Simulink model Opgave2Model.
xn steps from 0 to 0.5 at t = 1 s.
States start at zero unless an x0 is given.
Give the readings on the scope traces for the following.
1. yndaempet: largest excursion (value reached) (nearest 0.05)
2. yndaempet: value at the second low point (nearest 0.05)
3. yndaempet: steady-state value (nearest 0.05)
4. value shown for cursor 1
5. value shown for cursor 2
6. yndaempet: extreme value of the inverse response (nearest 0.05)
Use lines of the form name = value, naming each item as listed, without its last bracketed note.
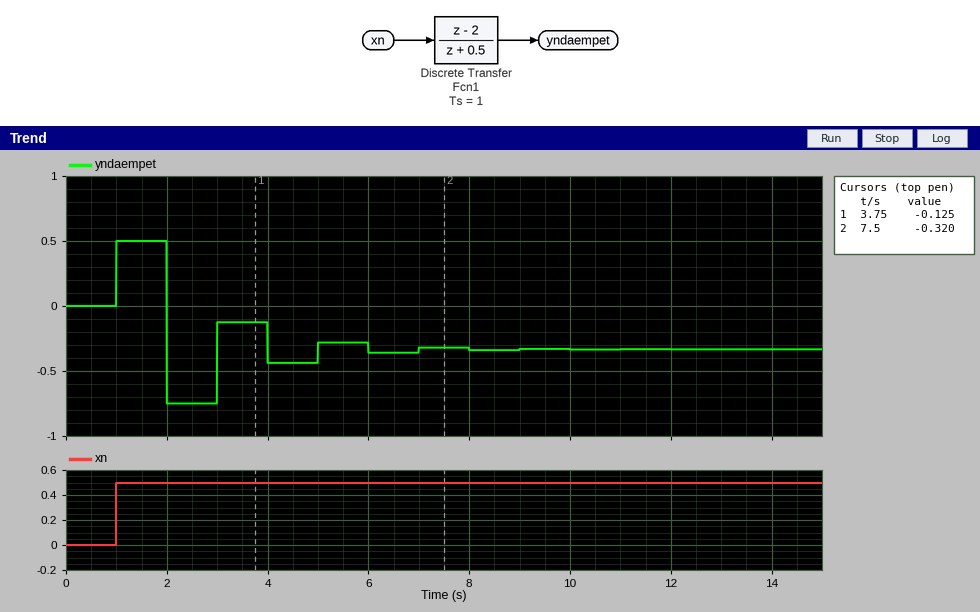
yndaempet: largest excursion (value reached) = -0.75
yndaempet: value at the second low point = -0.45
yndaempet: steady-state value = -0.35
value shown for cursor 1 = -0.125
value shown for cursor 2 = -0.320
yndaempet: extreme value of the inverse response = 0.50
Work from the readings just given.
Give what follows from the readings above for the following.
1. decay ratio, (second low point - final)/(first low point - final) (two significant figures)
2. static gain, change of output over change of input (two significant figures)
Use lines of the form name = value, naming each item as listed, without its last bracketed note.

decay ratio, (second low point - final)/(first low point - final) = 0.25
static gain, change of output over change of input = -0.70
